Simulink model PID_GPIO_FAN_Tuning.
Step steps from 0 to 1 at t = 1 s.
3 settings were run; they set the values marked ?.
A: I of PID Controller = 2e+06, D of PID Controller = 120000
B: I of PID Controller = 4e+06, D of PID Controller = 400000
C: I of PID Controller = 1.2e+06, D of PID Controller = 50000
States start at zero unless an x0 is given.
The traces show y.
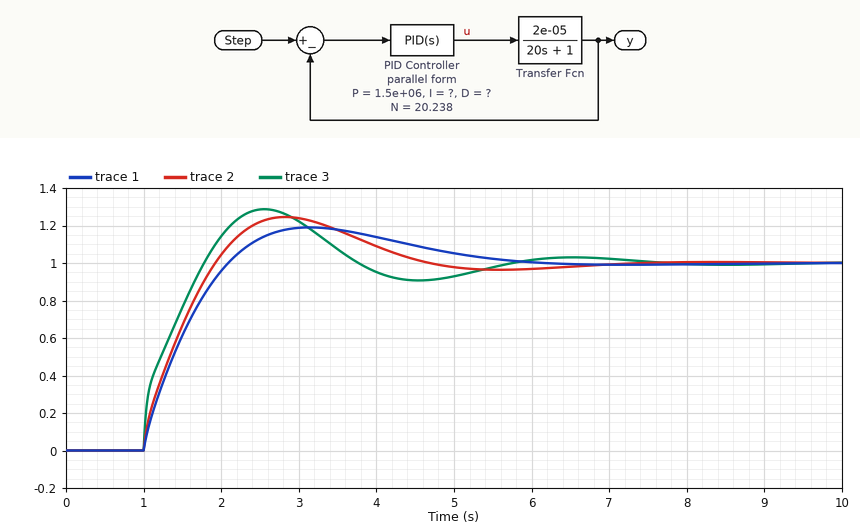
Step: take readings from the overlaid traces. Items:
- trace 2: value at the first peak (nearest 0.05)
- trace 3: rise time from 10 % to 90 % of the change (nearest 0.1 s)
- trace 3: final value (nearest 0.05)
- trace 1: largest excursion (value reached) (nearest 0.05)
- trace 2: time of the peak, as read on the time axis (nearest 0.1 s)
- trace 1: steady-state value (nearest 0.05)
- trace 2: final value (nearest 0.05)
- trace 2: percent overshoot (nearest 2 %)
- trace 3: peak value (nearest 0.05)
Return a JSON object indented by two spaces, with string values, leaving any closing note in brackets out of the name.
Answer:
{
  "trace 2: value at the first peak": "1.25",
  "trace 3: rise time from 10 % to 90 % of the change": "0.6 s",
  "trace 3: final value": "1.00",
  "trace 1: largest excursion (value reached)": "1.20",
  "trace 2: time of the peak, as read on the time axis": "2.8 s",
  "trace 1: steady-state value": "1.00",
  "trace 2: final value": "1.00",
  "trace 2: percent overshoot": "24 %",
  "trace 3: peak value": "1.30"
}
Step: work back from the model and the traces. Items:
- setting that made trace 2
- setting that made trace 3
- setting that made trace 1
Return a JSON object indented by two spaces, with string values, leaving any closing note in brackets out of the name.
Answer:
{
  "setting that made trace 2": "A",
  "setting that made trace 3": "B",
  "setting that made trace 1": "C"
}
